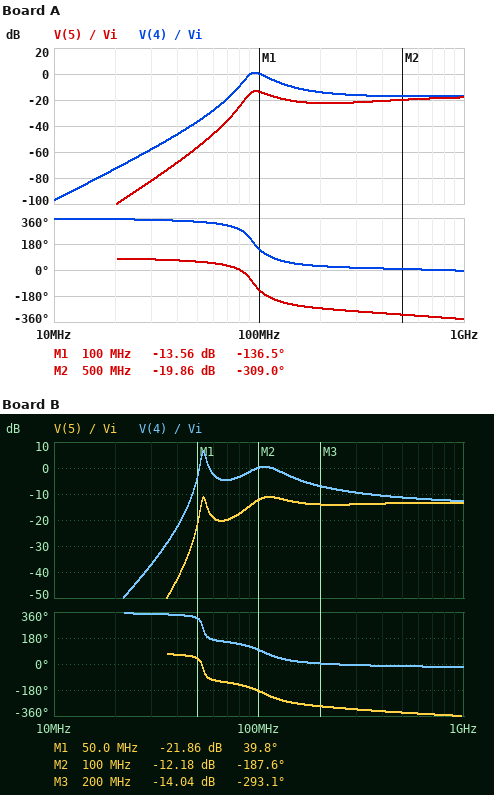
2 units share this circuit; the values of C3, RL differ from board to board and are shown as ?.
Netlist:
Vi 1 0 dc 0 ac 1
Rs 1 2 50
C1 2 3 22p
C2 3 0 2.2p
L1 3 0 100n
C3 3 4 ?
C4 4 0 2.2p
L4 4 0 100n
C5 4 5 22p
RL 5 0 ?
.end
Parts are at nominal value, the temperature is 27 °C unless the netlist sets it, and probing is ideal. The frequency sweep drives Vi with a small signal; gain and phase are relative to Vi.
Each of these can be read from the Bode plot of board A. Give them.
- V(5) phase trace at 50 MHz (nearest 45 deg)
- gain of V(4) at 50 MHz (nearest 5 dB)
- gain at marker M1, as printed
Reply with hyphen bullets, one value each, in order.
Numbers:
- 45 deg
- -35 dB
- -13.56 dB
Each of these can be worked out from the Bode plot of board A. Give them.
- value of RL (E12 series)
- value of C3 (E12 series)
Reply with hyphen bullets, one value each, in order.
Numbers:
- 15 Ω
- 3.9 pF
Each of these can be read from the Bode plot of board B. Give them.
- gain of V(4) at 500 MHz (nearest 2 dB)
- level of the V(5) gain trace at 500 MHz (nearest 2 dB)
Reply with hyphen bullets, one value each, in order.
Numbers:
- -12 dB
- -14 dB
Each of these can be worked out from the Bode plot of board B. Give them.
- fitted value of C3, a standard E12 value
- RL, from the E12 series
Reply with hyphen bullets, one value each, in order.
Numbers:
- 33 pF
- 18 Ω
